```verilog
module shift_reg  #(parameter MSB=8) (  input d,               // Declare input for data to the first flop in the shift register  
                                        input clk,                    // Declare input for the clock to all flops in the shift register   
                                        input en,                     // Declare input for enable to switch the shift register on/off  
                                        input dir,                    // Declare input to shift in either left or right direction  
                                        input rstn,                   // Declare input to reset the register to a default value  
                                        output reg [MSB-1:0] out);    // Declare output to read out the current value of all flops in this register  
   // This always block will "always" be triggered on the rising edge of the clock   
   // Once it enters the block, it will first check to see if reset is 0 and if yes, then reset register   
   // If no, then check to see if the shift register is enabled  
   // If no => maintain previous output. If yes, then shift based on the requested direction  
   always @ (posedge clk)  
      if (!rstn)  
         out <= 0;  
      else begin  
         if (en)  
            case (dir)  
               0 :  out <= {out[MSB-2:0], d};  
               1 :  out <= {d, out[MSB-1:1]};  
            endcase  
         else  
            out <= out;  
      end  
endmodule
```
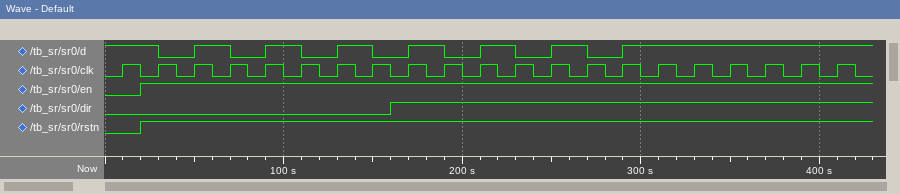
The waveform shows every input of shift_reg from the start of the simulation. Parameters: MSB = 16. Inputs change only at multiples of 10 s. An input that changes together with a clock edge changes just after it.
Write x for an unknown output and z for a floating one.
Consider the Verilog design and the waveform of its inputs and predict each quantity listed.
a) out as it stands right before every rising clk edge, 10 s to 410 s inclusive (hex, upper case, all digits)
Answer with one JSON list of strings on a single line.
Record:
["x, 0000, 0001, 0002, 0005, 000A, 0015, 002A, 0055, 002A, 8015, 400A, A005, 5002, A801, 5400, AA00, D500, EA80, F540, FAA0"]
